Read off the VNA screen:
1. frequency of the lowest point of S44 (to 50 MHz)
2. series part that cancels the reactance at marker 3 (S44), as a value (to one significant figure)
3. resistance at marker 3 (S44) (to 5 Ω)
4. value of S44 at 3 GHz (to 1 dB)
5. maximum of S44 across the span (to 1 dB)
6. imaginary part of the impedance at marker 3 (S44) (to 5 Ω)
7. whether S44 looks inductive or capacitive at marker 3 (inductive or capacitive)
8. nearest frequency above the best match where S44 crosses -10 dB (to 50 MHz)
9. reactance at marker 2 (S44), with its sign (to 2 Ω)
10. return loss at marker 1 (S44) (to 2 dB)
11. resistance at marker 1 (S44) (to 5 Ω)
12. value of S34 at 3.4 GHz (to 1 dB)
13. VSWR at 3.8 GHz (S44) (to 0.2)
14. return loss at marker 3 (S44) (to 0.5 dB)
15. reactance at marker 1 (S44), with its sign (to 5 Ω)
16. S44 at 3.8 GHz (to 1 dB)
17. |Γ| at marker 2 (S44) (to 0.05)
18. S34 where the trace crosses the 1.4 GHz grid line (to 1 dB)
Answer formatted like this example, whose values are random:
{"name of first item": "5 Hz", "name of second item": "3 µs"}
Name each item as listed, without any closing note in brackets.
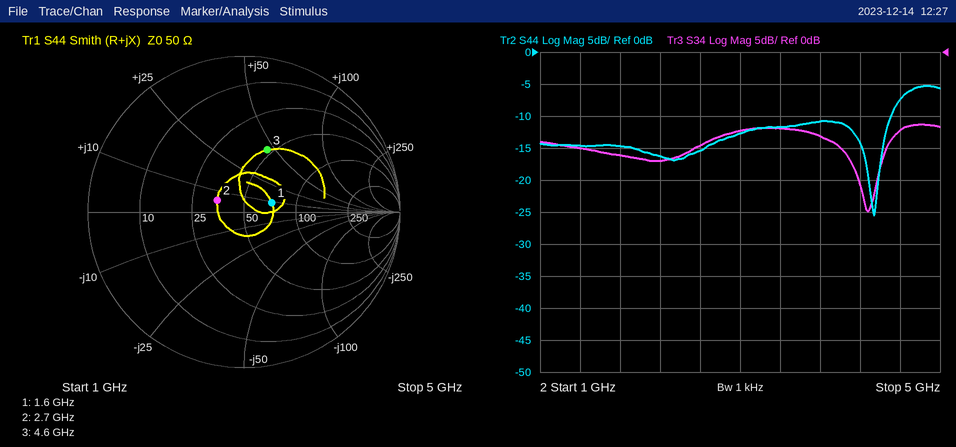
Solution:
{"frequency of the lowest point of S44": "4.35 GHz", "series part that cancels the reactance at marker 3 (S44), as a value": "800 fF", "resistance at marker 3 (S44)": "45 Ω", "value of S44 at 3 GHz": "-13 dB", "maximum of S44 across the span": "-5 dB", "imaginary part of the impedance at marker 3 (S44)": "+45 Ω", "whether S44 looks inductive or capacitive at marker 3": "inductive", "nearest frequency above the best match where S44 crosses -10 dB": "4.50 GHz", "reactance at marker 2 (S44), with its sign": "+6 Ω", "return loss at marker 1 (S44)": "14 dB", "resistance at marker 1 (S44)": "70 Ω", "value of S34 at 3.4 GHz": "-12 dB", "VSWR at 3.8 GHz (S44)": "1.8", "return loss at marker 3 (S44)": "7.5 dB", "reactance at marker 1 (S44), with its sign": "+10 Ω", "S44 at 3.8 GHz": "-11 dB", "|Γ| at marker 2 (S44)": "0.20", "S34 where the trace crosses the 1.4 GHz grid line": "-15 dB"}
